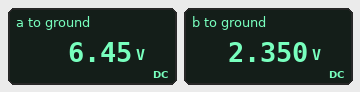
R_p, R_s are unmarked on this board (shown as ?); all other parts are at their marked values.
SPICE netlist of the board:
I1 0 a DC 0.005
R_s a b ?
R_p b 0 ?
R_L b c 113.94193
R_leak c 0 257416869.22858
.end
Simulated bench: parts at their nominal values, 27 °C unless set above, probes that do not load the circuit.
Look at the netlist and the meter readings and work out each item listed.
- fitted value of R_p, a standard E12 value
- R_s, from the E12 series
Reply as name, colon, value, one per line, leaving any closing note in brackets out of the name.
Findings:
fitted value of R_p, a standard E12 value: 470 Ω
R_s, from the E12 series: 820 Ω
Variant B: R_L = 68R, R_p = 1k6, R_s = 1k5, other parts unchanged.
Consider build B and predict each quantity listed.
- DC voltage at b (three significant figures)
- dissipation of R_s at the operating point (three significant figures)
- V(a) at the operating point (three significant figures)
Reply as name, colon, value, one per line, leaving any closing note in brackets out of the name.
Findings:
DC voltage at b: 8.00 V
dissipation of R_s at the operating point: 37.5 mW
V(a) at the operating point: 15.5 V
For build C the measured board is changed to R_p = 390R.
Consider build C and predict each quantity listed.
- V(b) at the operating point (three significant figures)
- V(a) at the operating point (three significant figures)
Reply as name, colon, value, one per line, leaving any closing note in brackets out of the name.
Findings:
V(b) at the operating point: 1.95 V
V(a) at the operating point: 6.05 V
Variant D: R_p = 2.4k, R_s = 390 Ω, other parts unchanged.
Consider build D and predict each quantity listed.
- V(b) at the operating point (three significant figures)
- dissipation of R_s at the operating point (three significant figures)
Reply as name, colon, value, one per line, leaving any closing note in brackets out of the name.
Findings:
V(b) at the operating point: 12.0 V
dissipation of R_s at the operating point: 9.75 mW
